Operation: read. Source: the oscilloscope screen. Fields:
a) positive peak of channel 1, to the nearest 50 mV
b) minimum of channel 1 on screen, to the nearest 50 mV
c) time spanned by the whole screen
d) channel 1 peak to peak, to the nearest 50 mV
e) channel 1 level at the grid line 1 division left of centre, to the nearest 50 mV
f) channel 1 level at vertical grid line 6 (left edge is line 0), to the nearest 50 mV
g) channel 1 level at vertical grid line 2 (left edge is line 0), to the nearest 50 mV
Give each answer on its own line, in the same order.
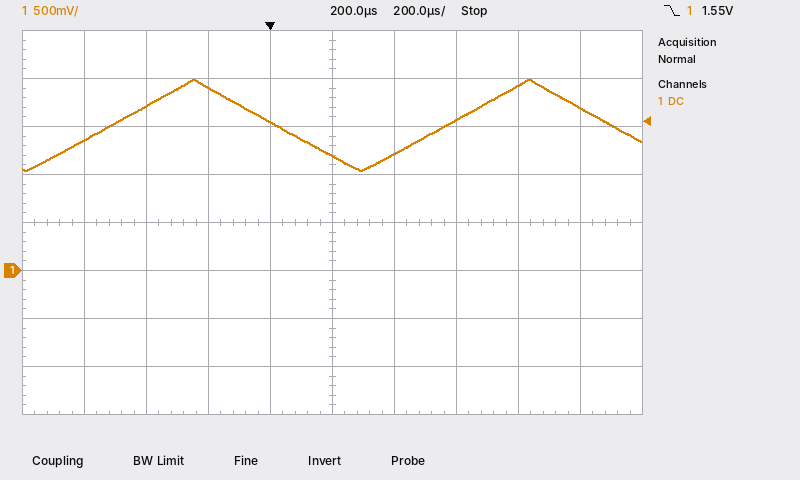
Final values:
2.00 V
1.05 V
2 ms
950 mV
1.55 V
1.20 V
1.70 V
